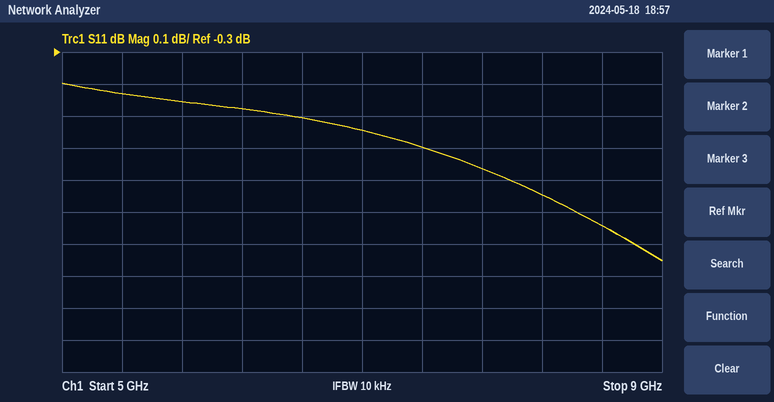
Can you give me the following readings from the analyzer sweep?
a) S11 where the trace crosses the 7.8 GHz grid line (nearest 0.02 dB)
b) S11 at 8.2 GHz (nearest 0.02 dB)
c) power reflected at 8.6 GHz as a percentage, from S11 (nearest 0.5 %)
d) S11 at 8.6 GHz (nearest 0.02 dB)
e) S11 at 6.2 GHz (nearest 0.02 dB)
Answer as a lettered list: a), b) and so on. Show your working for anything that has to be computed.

a) -0.66 dB
b) -0.74 dB
c) 10^(-0.84/10) ≈ 82.4 %, so 82.5 % to the nearest 0.5 %
d) -0.84 dB
e) -0.48 dB
